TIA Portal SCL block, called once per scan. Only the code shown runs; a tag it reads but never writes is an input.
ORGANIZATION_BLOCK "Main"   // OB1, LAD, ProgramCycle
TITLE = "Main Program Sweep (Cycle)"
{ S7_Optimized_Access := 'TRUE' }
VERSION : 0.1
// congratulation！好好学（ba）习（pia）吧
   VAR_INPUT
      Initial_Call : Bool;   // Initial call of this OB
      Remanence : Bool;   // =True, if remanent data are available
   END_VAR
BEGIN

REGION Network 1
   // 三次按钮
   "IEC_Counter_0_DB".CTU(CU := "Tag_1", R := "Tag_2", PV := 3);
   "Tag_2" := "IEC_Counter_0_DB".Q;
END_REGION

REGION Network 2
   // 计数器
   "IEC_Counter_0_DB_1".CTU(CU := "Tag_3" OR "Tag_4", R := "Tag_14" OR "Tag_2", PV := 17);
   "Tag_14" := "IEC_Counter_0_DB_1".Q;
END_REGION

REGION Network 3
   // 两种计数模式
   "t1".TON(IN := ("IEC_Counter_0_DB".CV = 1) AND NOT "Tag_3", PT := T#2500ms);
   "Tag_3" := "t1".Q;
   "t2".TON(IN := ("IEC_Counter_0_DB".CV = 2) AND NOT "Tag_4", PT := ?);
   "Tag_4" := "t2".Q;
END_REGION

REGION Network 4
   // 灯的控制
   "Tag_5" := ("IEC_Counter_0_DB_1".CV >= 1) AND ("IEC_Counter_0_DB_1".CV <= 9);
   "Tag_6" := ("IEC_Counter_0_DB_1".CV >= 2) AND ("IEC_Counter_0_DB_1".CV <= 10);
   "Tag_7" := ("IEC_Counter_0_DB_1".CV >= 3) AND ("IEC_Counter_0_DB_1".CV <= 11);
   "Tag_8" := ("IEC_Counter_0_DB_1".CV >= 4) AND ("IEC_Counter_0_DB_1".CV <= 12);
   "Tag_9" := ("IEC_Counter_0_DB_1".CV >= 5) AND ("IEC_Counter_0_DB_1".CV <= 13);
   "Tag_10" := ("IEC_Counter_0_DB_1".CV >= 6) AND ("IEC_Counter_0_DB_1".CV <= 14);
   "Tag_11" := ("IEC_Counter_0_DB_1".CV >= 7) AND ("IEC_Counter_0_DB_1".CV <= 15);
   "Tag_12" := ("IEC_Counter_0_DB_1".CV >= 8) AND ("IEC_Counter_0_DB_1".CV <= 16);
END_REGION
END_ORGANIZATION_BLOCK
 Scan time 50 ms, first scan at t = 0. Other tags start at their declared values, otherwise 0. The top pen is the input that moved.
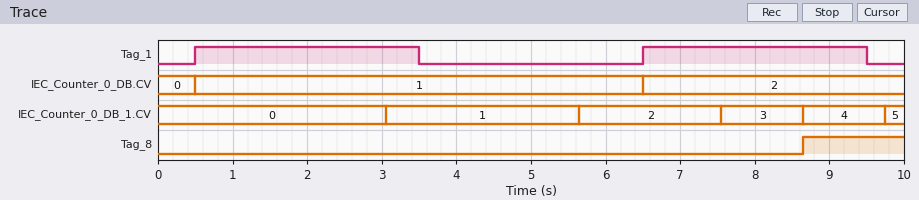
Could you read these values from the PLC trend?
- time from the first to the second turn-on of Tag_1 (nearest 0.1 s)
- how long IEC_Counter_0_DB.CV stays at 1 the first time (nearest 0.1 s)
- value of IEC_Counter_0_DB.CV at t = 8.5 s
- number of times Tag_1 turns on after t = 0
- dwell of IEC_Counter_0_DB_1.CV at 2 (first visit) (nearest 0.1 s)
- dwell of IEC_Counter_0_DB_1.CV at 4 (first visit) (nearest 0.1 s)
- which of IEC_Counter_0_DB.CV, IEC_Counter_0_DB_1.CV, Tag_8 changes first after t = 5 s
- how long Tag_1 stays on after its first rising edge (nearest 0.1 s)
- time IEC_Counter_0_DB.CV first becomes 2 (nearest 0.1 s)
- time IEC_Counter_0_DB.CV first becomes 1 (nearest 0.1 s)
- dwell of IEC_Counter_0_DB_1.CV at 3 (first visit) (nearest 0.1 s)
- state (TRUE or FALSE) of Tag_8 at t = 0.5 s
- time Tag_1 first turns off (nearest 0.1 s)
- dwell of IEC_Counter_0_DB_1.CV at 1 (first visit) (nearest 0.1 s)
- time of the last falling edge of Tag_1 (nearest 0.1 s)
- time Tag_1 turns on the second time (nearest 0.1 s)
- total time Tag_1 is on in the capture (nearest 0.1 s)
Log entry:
6.0 s
6.0 s
2
2
1.9 s
1.1 s
IEC_Counter_0_DB_1.CV
3.0 s
6.5 s
0.5 s
1.1 s
FALSE
3.5 s
2.6 s
9.5 s
6.5 s
6.0 s
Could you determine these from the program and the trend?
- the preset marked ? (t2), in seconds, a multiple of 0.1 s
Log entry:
1.0 s
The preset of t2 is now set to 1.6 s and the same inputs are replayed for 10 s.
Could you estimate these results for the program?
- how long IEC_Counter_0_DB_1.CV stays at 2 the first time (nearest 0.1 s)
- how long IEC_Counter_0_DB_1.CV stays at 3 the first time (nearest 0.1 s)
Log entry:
2.5 s
1.7 s
